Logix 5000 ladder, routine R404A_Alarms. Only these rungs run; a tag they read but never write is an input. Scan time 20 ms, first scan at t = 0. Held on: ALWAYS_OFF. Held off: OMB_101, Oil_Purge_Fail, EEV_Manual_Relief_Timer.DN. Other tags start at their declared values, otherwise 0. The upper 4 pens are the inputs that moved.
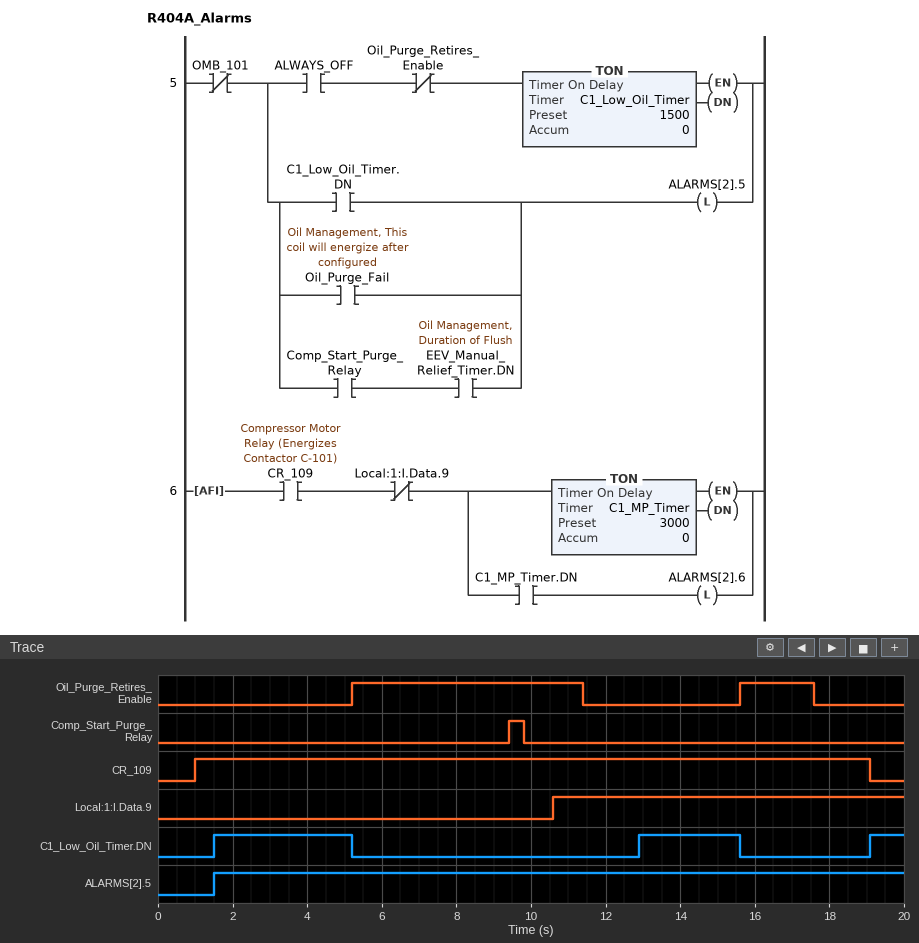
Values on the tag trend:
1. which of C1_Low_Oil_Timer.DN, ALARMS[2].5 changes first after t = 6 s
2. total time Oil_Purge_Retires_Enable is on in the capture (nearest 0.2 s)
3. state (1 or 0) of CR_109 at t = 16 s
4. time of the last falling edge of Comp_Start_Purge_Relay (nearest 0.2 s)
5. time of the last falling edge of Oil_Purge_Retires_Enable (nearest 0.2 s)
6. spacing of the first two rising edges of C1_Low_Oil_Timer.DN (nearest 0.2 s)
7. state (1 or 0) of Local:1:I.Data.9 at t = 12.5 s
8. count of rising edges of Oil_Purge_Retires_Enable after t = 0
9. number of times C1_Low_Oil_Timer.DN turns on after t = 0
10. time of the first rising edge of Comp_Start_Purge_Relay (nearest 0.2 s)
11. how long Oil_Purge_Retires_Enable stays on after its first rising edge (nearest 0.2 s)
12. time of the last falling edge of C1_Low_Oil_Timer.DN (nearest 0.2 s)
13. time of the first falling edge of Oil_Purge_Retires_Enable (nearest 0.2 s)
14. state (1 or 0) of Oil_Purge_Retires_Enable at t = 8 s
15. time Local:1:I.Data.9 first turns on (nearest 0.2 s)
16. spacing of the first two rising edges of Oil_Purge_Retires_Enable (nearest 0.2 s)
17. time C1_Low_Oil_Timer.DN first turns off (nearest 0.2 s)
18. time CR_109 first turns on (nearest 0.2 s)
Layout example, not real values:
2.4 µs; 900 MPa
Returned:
C1_Low_Oil_Timer.DN; 8.2 s; 1; 9.8 s; 17.6 s; 11.4 s; 1; 2; 3; 9.4 s; 6.2 s; 15.6 s; 11.4 s; 1; 10.6 s; 10.4 s; 5.2 s; 1.0 s
